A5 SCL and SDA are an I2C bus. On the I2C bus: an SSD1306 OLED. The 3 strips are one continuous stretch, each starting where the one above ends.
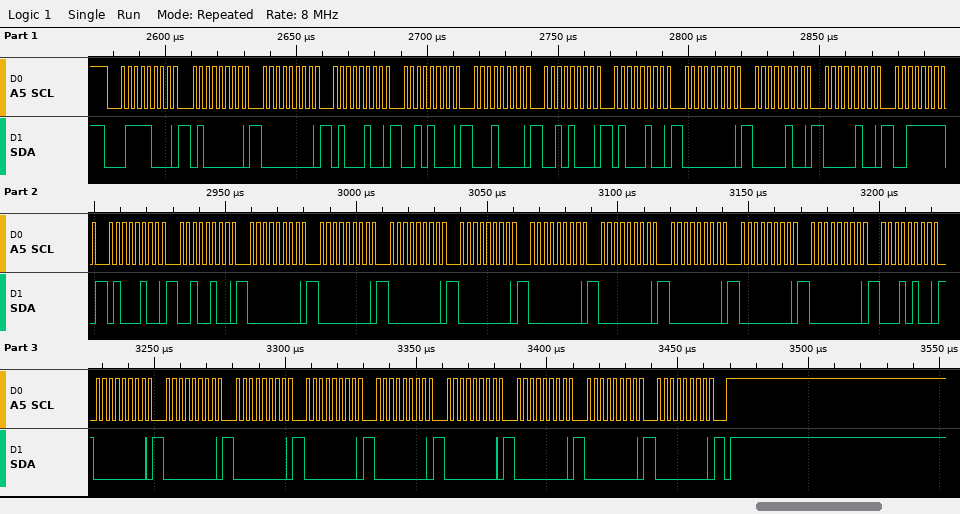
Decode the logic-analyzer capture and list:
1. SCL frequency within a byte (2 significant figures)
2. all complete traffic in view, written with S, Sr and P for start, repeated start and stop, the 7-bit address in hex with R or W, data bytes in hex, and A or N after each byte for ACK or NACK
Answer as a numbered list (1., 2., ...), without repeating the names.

1. 400 kHz
2. S 3CW A 40 A 00 A 44 A 28 A 10 A 28 A 44 A 00 A 04 A 04 A 3F A 44 A 24 A 00 A 00 A 00 A 00 A 00 A 00 A 00 A 00 A 00 A 14 A 00 A 00 A 00 A 00 A 00 A 00 A 00 A 00 A 00 A P
